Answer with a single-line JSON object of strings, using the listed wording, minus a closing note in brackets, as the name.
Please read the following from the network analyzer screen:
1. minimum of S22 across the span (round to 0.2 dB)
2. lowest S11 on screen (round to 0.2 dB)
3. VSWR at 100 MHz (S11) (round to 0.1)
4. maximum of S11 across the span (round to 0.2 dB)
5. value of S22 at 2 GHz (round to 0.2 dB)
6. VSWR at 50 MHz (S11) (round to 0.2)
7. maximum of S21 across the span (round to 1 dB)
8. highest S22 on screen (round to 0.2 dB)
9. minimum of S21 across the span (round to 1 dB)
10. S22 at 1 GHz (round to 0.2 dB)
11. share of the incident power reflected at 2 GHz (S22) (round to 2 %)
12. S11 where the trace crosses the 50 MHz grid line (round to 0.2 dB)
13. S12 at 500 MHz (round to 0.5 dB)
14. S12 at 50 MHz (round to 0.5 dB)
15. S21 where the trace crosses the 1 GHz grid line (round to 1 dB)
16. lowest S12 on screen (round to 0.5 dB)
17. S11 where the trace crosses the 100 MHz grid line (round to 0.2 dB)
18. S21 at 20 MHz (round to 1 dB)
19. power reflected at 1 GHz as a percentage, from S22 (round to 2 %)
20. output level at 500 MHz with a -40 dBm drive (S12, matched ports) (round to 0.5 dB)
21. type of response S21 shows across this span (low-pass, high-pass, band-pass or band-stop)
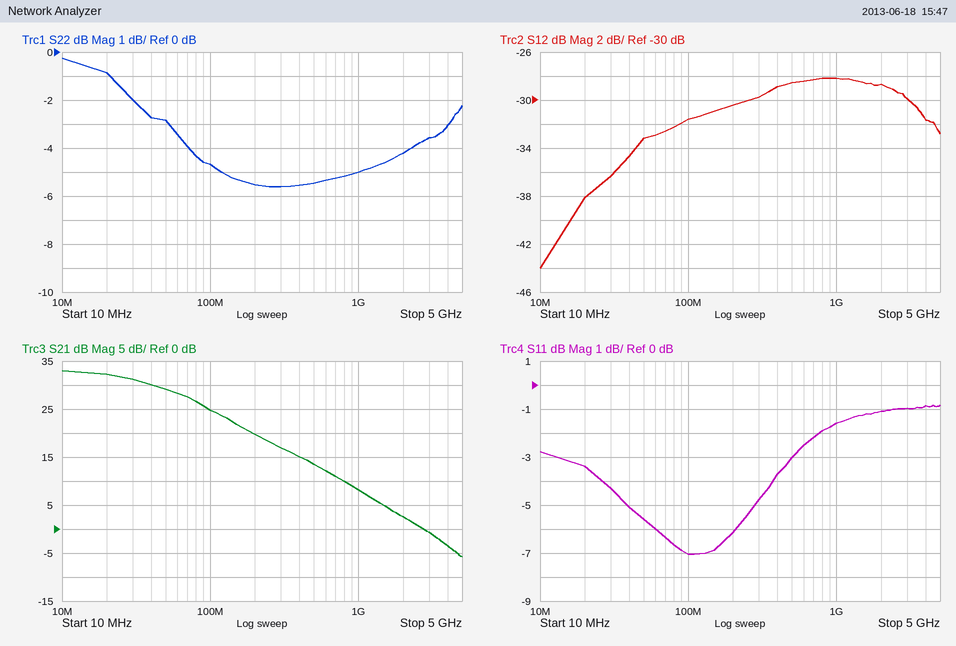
{"minimum of S22 across the span": "-5.6 dB", "lowest S11 on screen": "-7.0 dB", "VSWR at 100 MHz (S11)": "2.6", "maximum of S11 across the span": "-0.8 dB", "value of S22 at 2 GHz": "-4.2 dB", "VSWR at 50 MHz (S11)": "3.2", "maximum of S21 across the span": "33 dB", "highest S22 on screen": "-0.2 dB", "minimum of S21 across the span": "-6 dB", "S22 at 1 GHz": "-5.0 dB", "share of the incident power reflected at 2 GHz (S22)": "38 %", "S11 where the trace crosses the 50 MHz grid line": "-5.6 dB", "S12 at 500 MHz": "-28.5 dB", "S12 at 50 MHz": "-33.0 dB", "S21 where the trace crosses the 1 GHz grid line": "8 dB", "lowest S12 on screen": "-44.0 dB", "S11 where the trace crosses the 100 MHz grid line": "-7.0 dB", "S21 at 20 MHz": "32 dB", "power reflected at 1 GHz as a percentage, from S22": "32 %", "output level at 500 MHz with a -40 dBm drive (S12, matched ports)": "-68.5 dBm", "type of response S21 shows across this span": "low-pass"}
